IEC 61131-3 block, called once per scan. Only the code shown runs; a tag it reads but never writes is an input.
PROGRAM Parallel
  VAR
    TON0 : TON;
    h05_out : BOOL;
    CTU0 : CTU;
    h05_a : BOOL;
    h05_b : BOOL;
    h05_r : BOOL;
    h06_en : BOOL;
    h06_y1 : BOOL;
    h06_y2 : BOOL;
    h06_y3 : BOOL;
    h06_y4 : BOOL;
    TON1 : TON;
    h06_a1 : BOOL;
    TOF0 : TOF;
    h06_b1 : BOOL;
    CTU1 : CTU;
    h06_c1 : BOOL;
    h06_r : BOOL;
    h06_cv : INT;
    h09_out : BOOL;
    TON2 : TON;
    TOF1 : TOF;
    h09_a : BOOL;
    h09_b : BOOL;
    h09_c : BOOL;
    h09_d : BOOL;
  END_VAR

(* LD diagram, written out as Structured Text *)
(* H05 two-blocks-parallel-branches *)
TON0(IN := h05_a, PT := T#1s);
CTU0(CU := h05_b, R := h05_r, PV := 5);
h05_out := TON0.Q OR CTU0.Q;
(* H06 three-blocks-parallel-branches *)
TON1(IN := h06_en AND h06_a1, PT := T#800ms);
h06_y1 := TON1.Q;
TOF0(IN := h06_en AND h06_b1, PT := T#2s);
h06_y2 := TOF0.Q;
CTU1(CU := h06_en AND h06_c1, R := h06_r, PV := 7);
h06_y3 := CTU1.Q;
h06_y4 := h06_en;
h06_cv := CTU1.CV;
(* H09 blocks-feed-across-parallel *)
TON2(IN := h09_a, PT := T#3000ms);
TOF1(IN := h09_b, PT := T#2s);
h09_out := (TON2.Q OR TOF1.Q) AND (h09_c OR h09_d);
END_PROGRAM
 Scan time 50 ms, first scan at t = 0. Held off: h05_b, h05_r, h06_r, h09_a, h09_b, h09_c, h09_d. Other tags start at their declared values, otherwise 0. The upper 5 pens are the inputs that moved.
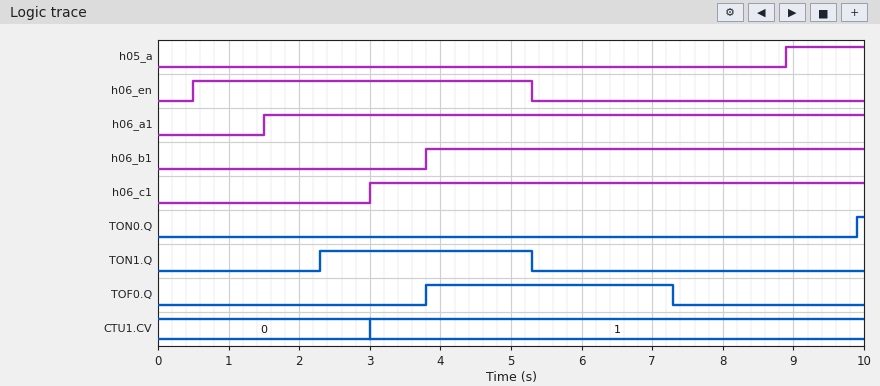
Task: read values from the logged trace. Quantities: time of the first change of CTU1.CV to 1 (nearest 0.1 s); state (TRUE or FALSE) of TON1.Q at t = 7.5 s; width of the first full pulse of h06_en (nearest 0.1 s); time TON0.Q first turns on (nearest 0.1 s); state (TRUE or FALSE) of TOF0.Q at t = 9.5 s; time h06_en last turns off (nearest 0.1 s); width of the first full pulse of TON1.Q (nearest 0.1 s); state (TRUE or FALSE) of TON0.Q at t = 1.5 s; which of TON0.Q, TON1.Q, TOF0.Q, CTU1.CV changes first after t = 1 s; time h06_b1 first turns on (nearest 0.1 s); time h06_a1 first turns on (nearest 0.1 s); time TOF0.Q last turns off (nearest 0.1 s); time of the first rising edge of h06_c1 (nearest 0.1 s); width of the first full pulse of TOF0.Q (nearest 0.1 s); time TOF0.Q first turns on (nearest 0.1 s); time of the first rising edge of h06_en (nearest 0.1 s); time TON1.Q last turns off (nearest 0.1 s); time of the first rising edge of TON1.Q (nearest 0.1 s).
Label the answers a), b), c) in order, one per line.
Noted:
a) 3.0 s
b) FALSE
c) 4.8 s
d) 9.9 s
e) FALSE
f) 5.3 s
g) 3.0 s
h) FALSE
i) TON1.Q
j) 3.8 s
k) 1.5 s
l) 7.3 s
m) 3.0 s
n) 3.5 s
o) 3.8 s
p) 0.5 s
q) 5.3 s
r) 2.3 s
